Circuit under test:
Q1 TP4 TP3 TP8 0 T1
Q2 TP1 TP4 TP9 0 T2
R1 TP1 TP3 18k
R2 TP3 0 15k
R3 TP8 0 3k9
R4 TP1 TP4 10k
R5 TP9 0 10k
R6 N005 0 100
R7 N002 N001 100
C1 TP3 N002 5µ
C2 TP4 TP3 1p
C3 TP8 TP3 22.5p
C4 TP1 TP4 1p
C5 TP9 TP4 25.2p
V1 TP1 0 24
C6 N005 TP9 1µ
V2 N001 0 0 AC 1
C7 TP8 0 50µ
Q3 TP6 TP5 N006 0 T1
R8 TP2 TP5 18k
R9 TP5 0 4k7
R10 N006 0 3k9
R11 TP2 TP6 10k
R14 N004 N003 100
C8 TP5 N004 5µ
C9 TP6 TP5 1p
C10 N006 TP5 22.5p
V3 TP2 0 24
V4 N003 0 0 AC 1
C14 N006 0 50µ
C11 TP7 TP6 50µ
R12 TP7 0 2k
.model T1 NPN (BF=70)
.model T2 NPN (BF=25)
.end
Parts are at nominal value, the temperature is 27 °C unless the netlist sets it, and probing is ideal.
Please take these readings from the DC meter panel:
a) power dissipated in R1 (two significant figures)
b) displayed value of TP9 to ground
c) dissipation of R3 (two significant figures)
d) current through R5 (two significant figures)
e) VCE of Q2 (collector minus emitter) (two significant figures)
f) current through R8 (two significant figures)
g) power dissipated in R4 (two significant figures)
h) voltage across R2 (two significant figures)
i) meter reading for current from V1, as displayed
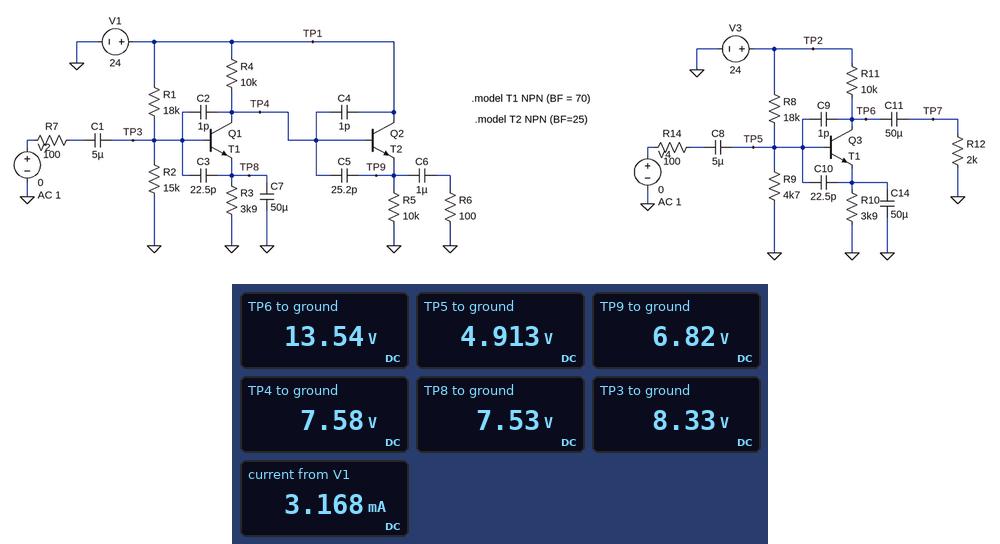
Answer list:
14 mW
6.82 V
15 mW
680 µA
17 V
1.1 mA
27 mW
8.3 V
3.168 mA
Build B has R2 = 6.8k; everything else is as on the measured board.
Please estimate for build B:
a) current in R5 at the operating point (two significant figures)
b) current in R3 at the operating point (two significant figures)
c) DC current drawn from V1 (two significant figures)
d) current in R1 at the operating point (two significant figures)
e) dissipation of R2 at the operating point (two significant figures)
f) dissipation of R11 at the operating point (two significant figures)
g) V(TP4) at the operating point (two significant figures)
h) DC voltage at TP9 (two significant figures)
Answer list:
850 µA
1.5 mA
3.3 mA
970 µA
6.2 mW
11 mW
9.3 V
8.5 V
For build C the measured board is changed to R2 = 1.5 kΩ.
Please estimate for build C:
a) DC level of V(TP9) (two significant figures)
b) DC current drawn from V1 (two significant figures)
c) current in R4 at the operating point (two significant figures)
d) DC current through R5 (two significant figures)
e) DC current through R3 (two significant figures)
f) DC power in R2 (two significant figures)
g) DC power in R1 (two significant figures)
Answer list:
20 V
3.5 mA
350 µA
2.0 mA
280 µA
2.3 mW
27 mW
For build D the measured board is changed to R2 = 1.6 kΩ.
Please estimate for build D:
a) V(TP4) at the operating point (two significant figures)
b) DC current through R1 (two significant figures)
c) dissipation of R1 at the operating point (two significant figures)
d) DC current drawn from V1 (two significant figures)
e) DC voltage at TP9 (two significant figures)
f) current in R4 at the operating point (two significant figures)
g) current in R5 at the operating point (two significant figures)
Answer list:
20 V
1.2 mA
27 mW
3.5 mA
19 V
380 µA
1.9 mA
